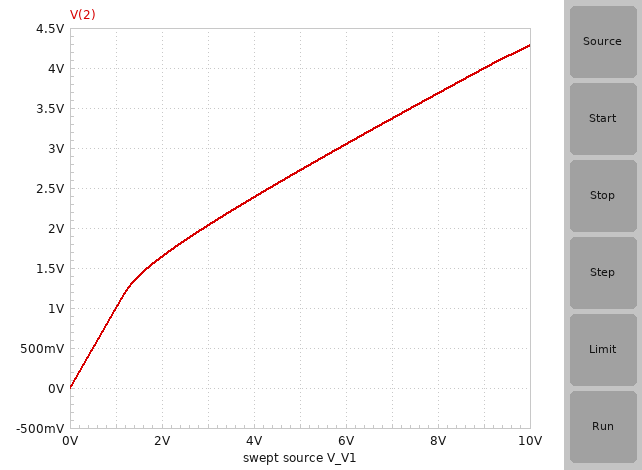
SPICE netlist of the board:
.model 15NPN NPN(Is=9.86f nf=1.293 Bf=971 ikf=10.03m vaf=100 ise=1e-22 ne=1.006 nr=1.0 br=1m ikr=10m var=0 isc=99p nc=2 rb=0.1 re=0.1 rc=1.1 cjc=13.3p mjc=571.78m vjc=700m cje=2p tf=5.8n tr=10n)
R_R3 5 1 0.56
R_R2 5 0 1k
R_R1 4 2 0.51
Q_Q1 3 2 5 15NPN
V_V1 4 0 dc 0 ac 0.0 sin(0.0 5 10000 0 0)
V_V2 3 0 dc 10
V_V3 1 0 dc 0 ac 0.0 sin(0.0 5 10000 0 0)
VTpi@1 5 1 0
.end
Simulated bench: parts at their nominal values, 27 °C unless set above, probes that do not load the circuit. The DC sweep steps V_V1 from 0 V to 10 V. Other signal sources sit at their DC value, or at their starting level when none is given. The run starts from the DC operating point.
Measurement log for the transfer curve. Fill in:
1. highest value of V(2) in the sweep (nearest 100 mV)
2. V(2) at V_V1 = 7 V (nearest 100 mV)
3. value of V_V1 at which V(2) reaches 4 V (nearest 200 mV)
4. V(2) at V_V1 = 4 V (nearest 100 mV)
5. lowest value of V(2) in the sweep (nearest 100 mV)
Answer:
4.3 V
3.4 V
9.0 V
2.4 V
0 V
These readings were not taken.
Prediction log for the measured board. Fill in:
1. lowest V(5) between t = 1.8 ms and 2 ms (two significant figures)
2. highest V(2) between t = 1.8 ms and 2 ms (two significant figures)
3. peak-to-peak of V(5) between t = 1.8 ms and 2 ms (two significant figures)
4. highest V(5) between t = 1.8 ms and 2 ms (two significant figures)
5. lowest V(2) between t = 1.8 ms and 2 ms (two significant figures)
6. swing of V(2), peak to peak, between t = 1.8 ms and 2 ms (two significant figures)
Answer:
-5.0 V
5.0 V
10 V
5.0 V
-5.0 V
10 V
